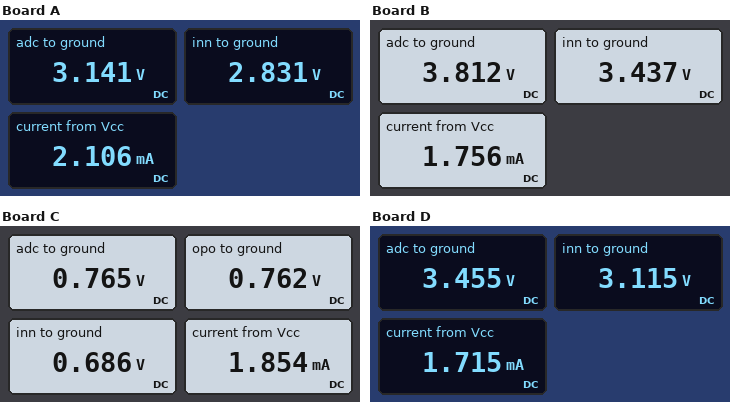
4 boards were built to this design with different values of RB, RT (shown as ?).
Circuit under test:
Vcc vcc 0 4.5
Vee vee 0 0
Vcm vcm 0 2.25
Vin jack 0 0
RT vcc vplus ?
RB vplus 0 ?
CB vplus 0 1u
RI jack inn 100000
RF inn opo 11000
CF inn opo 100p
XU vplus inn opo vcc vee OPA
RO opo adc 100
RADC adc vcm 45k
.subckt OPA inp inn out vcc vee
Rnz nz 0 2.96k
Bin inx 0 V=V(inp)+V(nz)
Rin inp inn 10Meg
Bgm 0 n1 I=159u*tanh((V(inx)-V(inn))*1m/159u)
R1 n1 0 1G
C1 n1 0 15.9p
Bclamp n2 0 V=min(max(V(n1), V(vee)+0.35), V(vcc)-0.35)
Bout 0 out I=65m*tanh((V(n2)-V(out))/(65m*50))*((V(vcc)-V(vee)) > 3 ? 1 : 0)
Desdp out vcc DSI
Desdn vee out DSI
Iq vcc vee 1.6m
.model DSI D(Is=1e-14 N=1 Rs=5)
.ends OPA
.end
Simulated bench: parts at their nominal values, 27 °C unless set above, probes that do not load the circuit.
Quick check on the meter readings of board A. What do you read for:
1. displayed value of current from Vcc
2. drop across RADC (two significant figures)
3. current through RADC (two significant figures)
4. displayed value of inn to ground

2.106 mA
890 mV
20 µA
2.831 V
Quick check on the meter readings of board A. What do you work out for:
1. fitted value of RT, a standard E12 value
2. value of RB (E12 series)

3.3 kΩ
5.6 kΩ
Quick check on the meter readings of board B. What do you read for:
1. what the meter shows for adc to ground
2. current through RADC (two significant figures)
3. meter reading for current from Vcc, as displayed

3.812 V
35 µA
1.756 mA
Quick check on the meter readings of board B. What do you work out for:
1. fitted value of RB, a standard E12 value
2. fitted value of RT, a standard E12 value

22 kΩ
6.8 kΩ
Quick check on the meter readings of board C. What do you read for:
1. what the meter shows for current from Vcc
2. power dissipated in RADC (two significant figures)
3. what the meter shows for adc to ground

1.854 mA
49 µW
0.765 V
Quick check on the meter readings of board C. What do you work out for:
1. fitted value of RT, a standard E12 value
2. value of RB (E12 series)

15 kΩ
2.7 kΩ
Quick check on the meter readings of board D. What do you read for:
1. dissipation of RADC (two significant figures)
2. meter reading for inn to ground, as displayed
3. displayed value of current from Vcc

32 µW
3.115 V
1.715 mA
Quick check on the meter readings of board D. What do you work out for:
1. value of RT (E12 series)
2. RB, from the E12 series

12 kΩ
27 kΩ
